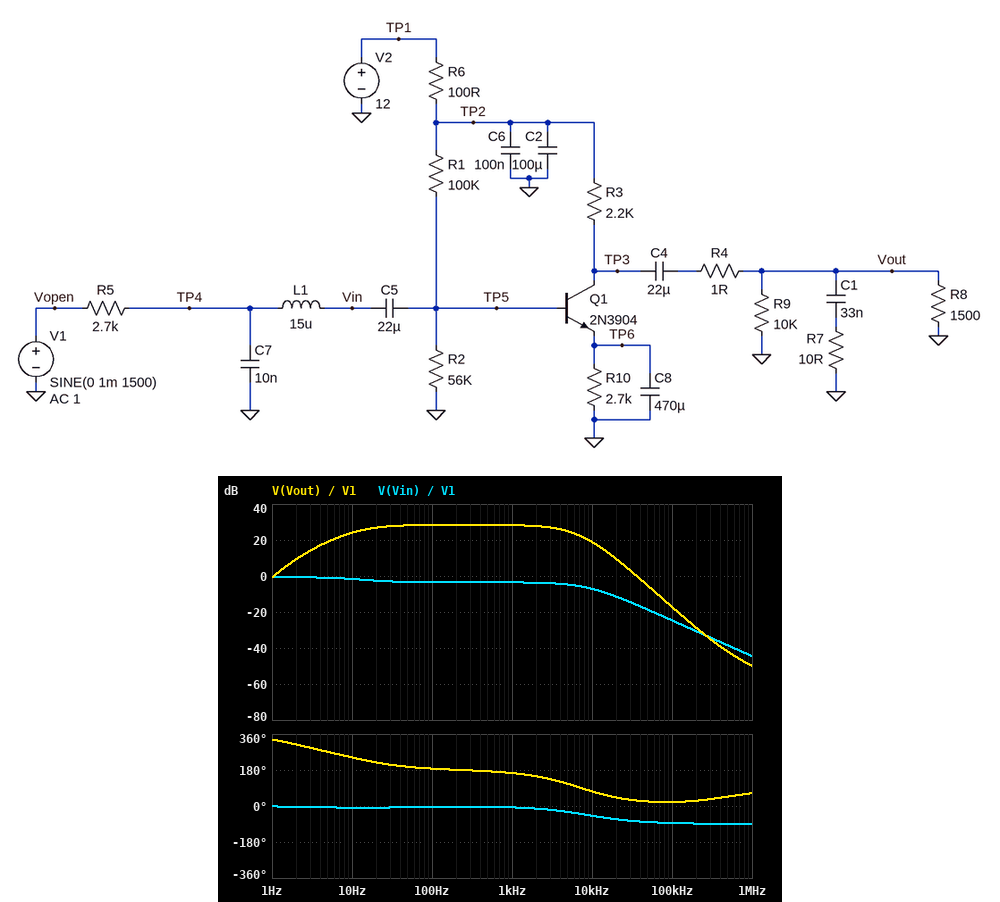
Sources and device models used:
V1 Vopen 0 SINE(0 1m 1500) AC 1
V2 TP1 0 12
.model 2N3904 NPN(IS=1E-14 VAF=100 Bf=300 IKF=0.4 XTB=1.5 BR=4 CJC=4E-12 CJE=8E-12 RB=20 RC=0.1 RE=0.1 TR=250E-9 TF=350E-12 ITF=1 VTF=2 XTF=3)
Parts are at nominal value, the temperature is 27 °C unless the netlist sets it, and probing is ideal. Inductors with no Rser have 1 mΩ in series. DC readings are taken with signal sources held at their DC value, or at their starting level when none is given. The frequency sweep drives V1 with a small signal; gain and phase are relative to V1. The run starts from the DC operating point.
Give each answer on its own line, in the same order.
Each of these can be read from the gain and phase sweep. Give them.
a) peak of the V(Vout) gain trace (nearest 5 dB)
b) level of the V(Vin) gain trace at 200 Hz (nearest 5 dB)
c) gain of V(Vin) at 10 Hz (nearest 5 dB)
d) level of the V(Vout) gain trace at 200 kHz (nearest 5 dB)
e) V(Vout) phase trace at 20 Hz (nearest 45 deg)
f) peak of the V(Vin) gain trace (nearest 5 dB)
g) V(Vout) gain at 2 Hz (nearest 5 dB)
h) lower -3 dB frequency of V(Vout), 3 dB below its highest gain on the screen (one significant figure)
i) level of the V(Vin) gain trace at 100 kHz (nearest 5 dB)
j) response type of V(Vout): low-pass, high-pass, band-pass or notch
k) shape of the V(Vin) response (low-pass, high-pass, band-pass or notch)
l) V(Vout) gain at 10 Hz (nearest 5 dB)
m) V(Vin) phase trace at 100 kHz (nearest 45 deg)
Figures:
30 dB
-5 dB
0 dB
-30 dB
225 deg
0 dB
10 dB
10 Hz
-25 dB
band-pass
low-pass
25 dB
-90 deg
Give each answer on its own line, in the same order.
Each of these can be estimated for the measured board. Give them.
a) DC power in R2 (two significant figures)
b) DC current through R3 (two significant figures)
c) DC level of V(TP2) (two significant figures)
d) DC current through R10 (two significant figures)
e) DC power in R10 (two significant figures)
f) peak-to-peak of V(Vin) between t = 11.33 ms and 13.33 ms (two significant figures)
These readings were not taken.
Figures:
300 µW
1.3 mA
12 V
1.3 mA
4.4 mW
1.3 mV
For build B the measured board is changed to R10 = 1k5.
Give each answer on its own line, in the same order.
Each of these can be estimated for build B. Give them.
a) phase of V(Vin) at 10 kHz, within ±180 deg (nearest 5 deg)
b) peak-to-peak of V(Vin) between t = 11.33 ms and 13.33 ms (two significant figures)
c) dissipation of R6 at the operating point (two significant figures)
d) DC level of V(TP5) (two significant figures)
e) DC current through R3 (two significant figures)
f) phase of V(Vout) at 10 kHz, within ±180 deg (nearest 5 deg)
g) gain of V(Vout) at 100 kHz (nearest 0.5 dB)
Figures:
-45 deg
1.1 mV
510 µW
4.0 V
2.2 mA
80 deg
-12.5 dB
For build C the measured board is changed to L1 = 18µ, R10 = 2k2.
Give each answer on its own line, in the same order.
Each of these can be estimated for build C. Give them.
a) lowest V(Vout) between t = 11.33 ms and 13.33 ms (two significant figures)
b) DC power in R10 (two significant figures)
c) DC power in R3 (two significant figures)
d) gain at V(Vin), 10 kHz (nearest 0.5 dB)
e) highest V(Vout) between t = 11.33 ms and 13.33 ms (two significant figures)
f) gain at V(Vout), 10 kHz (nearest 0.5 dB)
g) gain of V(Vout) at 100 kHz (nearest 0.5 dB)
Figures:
-29 mV
5.3 mW
5.2 mW
-7.5 dB
29 mV
20.5 dB
-15.5 dB
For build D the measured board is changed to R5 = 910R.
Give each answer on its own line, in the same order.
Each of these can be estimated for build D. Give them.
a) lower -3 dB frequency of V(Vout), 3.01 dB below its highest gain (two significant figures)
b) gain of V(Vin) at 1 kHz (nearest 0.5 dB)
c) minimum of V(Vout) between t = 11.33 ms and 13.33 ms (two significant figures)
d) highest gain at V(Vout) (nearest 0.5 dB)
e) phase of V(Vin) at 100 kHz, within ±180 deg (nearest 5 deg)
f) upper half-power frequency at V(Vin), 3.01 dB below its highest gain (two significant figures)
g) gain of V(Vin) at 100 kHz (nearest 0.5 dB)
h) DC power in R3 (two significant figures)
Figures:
16 Hz
-1.5 dB
-33 mV
30.5 dB
-80 deg
14 kHz
-15.5 dB
3.6 mW
